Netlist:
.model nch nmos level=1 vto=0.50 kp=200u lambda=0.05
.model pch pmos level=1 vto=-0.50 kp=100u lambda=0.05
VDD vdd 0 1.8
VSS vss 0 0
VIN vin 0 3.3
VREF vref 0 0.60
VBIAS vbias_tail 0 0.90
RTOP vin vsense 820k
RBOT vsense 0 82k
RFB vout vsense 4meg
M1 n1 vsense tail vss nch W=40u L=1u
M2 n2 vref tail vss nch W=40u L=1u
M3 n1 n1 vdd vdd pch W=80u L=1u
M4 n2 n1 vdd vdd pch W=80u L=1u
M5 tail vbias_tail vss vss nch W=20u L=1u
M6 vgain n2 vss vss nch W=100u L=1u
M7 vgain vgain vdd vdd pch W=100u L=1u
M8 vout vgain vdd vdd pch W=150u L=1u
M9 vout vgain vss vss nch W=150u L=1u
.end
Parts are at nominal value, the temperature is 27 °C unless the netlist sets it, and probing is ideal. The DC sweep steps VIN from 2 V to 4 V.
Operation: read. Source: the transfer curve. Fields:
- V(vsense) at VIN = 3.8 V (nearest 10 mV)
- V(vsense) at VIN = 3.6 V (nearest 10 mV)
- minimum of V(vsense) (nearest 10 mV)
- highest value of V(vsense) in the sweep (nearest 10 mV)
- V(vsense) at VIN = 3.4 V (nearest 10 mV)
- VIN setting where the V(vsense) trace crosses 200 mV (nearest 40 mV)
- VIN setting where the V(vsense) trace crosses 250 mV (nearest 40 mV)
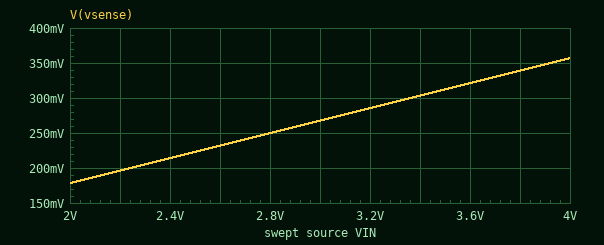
340 mV
320 mV
180 mV
360 mV
300 mV
2.24 V
2.80 V
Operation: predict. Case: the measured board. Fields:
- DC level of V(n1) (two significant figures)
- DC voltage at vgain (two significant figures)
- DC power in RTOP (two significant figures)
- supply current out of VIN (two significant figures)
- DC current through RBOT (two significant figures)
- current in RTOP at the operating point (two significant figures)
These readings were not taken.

1.3 V
1.3 V
11 µW
3.7 µA
3.6 µA
3.7 µA
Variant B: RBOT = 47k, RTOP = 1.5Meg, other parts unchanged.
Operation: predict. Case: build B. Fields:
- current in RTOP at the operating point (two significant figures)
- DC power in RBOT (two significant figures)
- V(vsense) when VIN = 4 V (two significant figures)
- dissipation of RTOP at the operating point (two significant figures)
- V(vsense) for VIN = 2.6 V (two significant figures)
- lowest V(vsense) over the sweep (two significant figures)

2.1 µA
210 nW
120 mV
6.8 µW
78 mV
60 mV
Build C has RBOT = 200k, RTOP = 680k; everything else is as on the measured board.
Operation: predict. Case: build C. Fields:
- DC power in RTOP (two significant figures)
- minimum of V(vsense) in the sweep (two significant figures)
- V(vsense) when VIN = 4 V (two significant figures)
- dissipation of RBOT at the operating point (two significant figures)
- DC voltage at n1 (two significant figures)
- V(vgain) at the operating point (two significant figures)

9.3 µW
440 mV
940 mV
3.1 µW
1.1 V
250 mV
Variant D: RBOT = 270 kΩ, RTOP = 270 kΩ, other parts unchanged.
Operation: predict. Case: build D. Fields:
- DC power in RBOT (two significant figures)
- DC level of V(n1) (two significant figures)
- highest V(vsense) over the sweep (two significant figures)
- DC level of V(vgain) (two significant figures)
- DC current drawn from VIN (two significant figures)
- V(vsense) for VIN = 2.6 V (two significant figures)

10 µW
1.0 V
2.0 V
250 mV
6.1 µA
1.3 V
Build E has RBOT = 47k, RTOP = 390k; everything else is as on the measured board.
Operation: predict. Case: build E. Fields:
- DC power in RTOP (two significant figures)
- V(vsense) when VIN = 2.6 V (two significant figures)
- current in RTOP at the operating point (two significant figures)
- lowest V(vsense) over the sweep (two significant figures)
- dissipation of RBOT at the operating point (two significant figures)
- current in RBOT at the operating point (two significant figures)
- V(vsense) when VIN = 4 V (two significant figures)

22 µW
280 mV
7.6 µA
210 mV
2.6 µW
7.5 µA
430 mV
